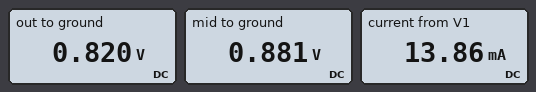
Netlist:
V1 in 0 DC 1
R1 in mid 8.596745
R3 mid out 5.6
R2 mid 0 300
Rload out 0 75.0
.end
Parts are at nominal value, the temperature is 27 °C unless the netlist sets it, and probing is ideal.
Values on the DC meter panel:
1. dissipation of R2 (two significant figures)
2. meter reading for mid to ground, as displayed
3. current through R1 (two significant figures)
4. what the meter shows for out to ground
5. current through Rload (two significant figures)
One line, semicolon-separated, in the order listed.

2.6 mW; 0.881 V; 14 mA; 0.820 V; 11 mA
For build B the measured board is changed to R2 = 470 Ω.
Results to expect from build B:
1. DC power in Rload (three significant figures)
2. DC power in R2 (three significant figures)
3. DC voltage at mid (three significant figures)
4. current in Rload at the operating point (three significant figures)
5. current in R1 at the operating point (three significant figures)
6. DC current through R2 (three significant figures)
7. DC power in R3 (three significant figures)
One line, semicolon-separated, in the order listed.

9.12 mW; 1.68 mW; 889 mV; 11.0 mA; 12.9 mA; 1.89 mA; 681 µW
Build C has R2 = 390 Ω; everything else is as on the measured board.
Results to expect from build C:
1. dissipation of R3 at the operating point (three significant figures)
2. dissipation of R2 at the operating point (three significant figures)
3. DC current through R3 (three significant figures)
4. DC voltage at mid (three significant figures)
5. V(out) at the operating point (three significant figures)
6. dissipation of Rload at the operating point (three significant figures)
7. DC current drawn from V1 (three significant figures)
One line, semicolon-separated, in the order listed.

677 µW; 2.01 mW; 11.0 mA; 886 mV; 824 mV; 9.06 mW; 13.3 mA
